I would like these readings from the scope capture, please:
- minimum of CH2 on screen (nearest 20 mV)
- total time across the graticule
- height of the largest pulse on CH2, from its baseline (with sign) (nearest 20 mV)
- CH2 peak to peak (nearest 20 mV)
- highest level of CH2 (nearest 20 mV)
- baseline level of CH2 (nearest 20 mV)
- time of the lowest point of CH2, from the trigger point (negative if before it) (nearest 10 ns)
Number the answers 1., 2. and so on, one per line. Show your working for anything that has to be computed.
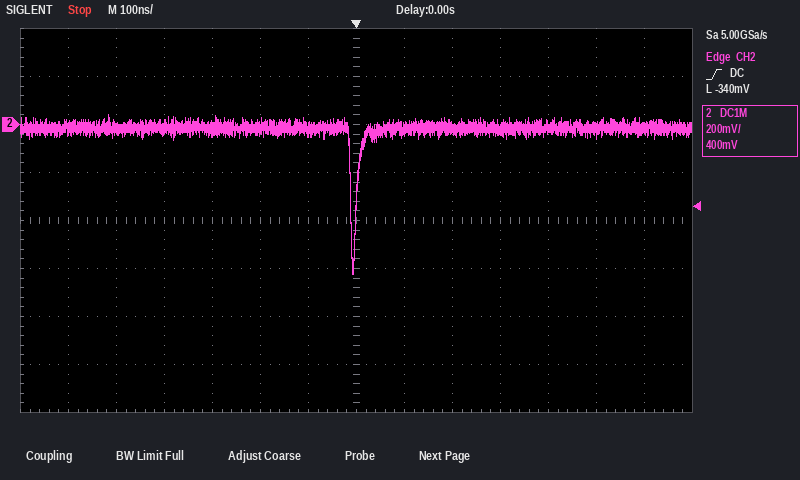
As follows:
1. -620 mV
2. 1.4 µs
3. -620 mV − (-20 mV) = -600 mV
4. 40 mV − (-620 mV) = 660 mV
5. 40 mV
6. -20 mV
7. -10 ns
